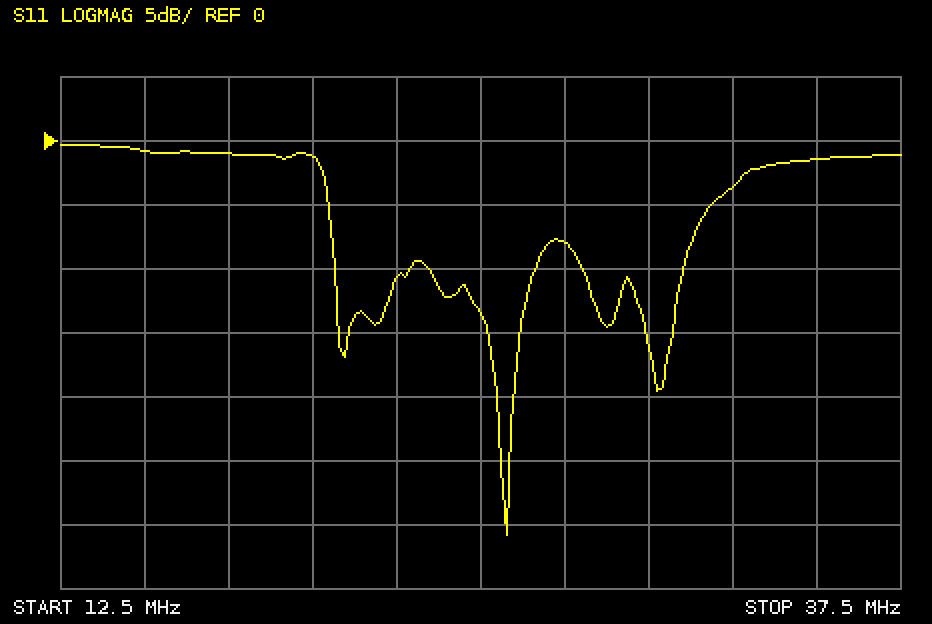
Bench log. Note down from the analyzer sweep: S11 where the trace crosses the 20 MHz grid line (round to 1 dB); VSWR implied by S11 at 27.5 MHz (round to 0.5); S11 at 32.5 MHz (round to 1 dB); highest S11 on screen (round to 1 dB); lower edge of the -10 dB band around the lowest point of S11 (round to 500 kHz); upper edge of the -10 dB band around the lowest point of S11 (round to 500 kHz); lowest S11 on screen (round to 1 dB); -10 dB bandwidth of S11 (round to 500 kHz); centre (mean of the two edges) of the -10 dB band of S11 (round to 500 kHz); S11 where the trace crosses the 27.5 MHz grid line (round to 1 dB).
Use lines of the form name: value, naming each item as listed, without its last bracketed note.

S11 where the trace crosses the 20 MHz grid line: -1 dB
VSWR implied by S11 at 27.5 MHz: 2.5
S11 at 32.5 MHz: -4 dB
highest S11 on screen: 0 dB
lower edge of the -10 dB band around the lowest point of S11: 23.5 MHz
upper edge of the -10 dB band around the lowest point of S11: 26.5 MHz
lowest S11 on screen: -31 dB
-10 dB bandwidth of S11: 3.0 MHz
centre (mean of the two edges) of the -10 dB band of S11: 25.0 MHz
S11 where the trace crosses the 27.5 MHz grid line: -8 dB
